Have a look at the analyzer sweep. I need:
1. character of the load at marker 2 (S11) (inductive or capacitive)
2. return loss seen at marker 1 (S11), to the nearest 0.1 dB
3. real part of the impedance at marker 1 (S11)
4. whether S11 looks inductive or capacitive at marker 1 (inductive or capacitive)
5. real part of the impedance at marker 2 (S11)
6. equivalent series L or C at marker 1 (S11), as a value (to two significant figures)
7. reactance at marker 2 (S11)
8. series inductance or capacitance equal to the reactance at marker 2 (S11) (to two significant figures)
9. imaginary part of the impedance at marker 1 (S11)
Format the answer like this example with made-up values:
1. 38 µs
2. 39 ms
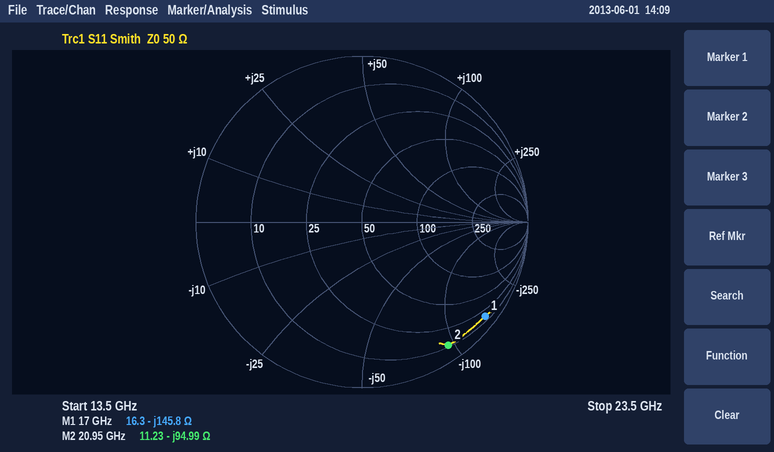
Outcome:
1. capacitive
2. 0.6 dB
3. 16.3 Ω
4. capacitive
5. 11.23 Ω
6. 64 fF
7. -94.99 Ω
8. 80 fF
9. -145.8 Ω
